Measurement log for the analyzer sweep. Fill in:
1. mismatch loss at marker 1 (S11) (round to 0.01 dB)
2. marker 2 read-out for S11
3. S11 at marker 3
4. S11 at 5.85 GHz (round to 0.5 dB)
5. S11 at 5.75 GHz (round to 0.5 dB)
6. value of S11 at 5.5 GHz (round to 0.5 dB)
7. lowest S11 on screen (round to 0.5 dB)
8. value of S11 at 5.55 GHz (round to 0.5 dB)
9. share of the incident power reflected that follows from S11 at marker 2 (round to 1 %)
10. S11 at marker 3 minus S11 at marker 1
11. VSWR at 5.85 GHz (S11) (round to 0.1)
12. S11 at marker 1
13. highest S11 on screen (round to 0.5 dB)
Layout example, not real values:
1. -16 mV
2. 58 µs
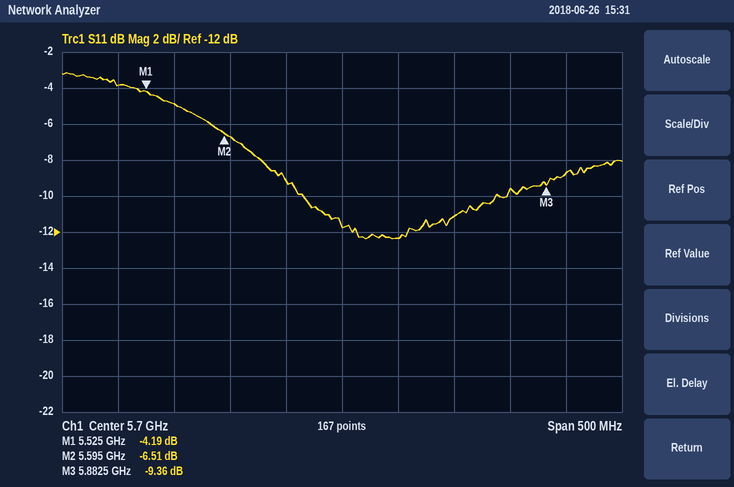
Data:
1. 2.08 dB
2. -6.51 dB
3. -9.36 dB
4. -9.5 dB
5. -12.5 dB
6. -4.0 dB
7. -12.5 dB
8. -5.0 dB
9. 22 %
10. -5.17 dB
11. 2.0
12. -4.19 dB
13. -3.0 dB
